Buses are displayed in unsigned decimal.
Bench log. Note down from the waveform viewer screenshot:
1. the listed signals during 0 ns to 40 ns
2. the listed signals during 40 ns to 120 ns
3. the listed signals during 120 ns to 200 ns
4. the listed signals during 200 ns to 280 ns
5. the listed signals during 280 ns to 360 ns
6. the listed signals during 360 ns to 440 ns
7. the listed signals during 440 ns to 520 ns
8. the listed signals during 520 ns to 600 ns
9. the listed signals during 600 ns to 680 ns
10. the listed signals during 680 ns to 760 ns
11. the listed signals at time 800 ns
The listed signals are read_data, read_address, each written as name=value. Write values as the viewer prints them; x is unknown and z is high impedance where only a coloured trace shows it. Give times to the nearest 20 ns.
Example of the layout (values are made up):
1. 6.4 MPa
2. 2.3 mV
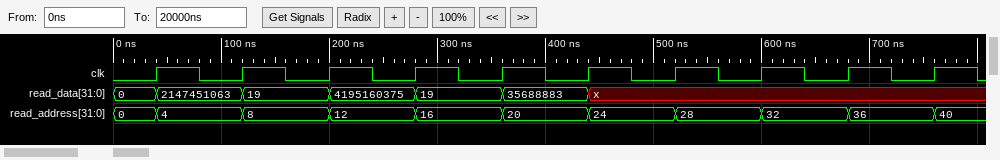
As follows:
1. read_data=0, read_address=0
2. read_data=2147451063, read_address=4
3. read_data=19, read_address=8
4. read_data=4195160375, read_address=12
5. read_data=19, read_address=16
6. read_data=35688883, read_address=20
7. read_data=x, read_address=24
8. read_data=x, read_address=28
9. read_data=x, read_address=32
10. read_data=x, read_address=36
11. read_data=x, read_address=40
